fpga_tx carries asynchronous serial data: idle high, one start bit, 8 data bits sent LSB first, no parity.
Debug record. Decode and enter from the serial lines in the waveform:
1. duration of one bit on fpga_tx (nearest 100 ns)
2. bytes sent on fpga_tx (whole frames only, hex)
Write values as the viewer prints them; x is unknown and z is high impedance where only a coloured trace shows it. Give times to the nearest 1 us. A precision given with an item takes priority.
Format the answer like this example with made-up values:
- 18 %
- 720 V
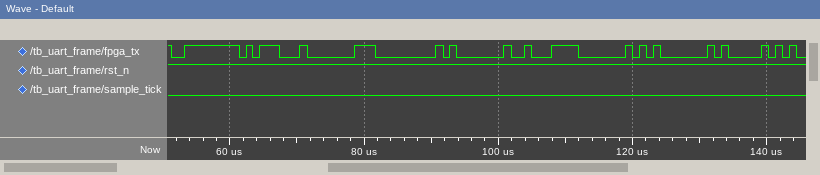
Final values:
- 1000 ns
- FE, 1D, C0, 00, 01, E2, 40, 01, 41
